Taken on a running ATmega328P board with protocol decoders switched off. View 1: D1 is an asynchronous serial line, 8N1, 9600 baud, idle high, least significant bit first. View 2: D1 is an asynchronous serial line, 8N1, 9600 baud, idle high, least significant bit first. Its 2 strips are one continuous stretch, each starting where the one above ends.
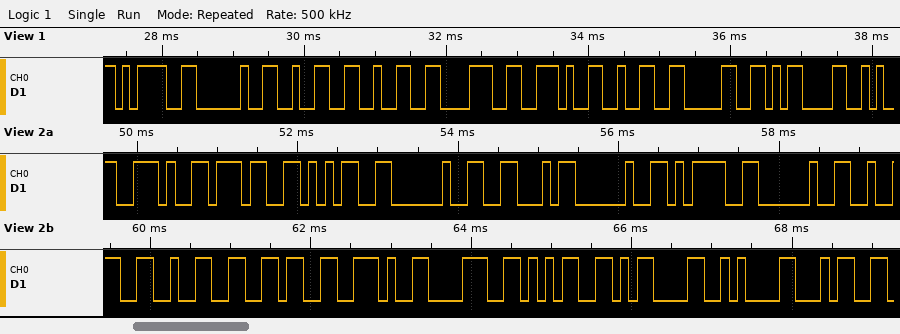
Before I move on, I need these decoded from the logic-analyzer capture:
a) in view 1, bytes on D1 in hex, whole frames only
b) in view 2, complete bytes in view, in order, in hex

3D 20 32 32 38 2E 32 30 0D
0x2E 0x37 0x35 0x20 0x46 0x20 0x3D 0x20 0x32 0x32 0x36 0x2E 0x38 0x35 0x0D 0x0A 0x34
